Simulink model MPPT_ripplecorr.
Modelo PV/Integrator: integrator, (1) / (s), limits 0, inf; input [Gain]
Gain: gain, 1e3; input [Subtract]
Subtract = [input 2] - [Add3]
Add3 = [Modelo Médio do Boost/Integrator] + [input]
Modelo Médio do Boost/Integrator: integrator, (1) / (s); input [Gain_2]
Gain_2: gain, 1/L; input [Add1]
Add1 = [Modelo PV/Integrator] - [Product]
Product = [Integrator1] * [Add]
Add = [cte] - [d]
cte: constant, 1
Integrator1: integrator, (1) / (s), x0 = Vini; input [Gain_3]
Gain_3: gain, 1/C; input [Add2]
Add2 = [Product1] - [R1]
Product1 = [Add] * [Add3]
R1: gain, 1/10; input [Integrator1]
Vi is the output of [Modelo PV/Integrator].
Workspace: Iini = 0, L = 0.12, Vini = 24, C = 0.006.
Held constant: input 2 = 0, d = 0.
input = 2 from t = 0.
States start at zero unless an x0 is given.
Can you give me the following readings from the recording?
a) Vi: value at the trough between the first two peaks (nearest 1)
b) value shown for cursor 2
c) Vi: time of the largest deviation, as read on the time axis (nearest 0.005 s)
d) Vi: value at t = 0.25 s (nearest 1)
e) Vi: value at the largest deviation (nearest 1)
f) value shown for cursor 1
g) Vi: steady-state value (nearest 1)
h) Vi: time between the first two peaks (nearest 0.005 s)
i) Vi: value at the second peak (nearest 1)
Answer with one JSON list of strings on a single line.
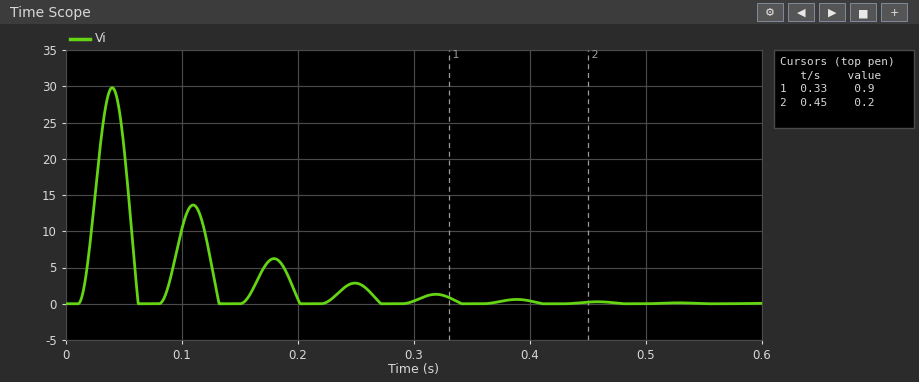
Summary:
["0", "0.2", "0.040 s", "3", "30", "0.9", "0", "0.070 s", "14"]
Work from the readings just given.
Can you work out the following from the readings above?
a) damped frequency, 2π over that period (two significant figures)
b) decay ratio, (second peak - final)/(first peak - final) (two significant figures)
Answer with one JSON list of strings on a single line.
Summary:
["90 rad/s", "0.47"]
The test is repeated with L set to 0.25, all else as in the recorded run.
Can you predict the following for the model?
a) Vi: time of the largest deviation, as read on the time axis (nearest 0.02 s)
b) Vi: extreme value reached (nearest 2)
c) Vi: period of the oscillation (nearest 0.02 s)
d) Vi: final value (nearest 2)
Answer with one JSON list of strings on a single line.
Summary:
["0.06 s", "24", "0.10 s", "0"]
